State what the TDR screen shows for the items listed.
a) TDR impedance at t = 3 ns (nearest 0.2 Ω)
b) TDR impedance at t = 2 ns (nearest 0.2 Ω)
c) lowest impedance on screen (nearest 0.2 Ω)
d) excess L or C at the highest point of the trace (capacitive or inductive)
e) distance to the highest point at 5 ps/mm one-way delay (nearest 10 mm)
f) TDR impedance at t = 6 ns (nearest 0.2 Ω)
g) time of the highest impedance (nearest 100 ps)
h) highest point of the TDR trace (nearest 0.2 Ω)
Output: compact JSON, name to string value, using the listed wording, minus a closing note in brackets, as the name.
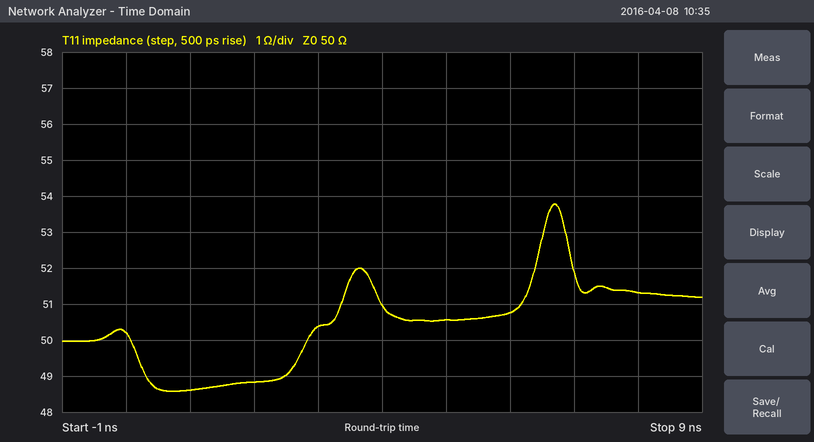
{"TDR impedance at t = 3 ns": "50.4 Ω", "TDR impedance at t = 2 ns": "48.8 Ω", "lowest impedance on screen": "48.6 Ω", "excess L or C at the highest point of the trace": "inductive", "distance to the highest point at 5 ps/mm one-way delay": "670 mm", "TDR impedance at t = 6 ns": "50.8 Ω", "time of the highest impedance": "6.7 ns", "highest point of the TDR trace": "53.8 Ω"}
